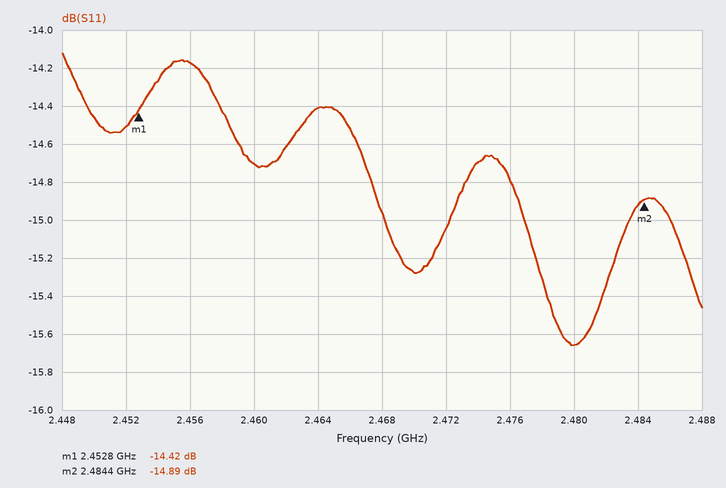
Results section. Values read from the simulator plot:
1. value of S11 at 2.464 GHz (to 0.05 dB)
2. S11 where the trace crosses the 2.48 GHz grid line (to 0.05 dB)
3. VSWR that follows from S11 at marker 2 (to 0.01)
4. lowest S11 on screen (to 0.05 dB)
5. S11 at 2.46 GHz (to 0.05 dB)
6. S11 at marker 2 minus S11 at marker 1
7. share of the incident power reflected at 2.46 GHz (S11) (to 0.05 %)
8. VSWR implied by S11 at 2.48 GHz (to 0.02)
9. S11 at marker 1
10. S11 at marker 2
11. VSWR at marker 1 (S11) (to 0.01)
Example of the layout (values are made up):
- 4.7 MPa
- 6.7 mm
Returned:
- -14.40 dB
- -15.65 dB
- 1.44
- -15.65 dB
- -14.70 dB
- -0.47 dB
- 3.40 %
- 1.40
- -14.42 dB
- -14.89 dB
- 1.47
